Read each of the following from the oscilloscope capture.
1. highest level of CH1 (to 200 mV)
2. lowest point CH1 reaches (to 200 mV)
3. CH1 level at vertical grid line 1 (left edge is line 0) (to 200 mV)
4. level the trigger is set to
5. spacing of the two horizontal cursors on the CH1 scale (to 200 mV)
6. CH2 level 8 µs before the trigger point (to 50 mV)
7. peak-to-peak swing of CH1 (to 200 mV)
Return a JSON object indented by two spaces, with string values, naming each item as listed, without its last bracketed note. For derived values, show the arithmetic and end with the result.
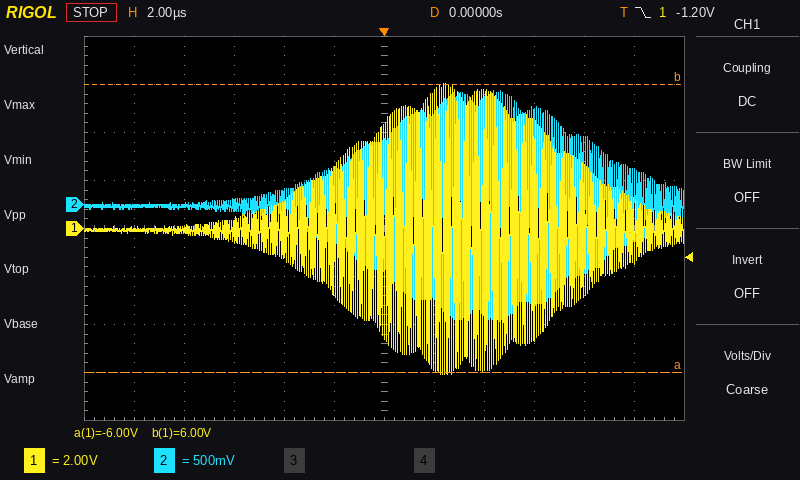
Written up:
{
  "highest level of CH1": "6.0 V",
  "lowest point CH1 reaches": "-6.0 V",
  "CH1 level at vertical grid line 1 (left edge is line 0)": "0.0 V",
  "level the trigger is set to": "-1.20 V",
  "spacing of the two horizontal cursors on the CH1 scale": "12.0 V",
  "CH2 level 8 µs before the trigger point": "0 mV",
  "peak-to-peak swing of CH1": "6.0 V − (-6.0 V) = 12.0 V"
}
